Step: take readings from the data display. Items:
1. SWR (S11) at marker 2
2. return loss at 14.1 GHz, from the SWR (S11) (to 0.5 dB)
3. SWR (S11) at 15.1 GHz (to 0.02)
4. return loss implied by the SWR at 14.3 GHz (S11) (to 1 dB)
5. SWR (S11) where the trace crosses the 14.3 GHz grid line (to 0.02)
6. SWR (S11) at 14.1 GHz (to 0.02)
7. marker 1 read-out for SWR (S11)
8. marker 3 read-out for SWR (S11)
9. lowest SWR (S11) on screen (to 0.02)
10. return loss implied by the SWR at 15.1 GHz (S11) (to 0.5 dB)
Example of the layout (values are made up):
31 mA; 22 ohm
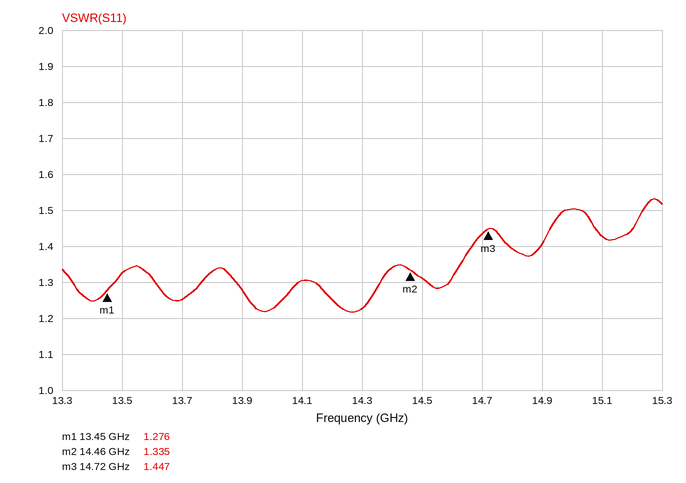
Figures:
1.335; 17.5 dB; 1.42; 20 dB; 1.22; 1.30; 1.276; 1.447; 1.22; 15.0 dB
